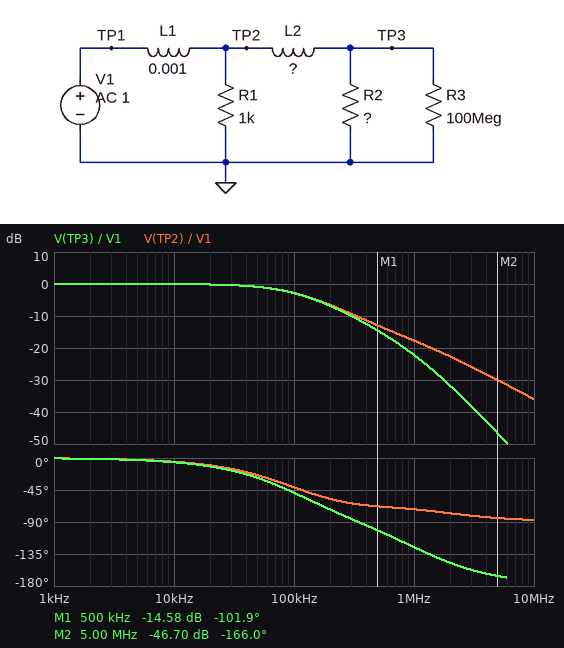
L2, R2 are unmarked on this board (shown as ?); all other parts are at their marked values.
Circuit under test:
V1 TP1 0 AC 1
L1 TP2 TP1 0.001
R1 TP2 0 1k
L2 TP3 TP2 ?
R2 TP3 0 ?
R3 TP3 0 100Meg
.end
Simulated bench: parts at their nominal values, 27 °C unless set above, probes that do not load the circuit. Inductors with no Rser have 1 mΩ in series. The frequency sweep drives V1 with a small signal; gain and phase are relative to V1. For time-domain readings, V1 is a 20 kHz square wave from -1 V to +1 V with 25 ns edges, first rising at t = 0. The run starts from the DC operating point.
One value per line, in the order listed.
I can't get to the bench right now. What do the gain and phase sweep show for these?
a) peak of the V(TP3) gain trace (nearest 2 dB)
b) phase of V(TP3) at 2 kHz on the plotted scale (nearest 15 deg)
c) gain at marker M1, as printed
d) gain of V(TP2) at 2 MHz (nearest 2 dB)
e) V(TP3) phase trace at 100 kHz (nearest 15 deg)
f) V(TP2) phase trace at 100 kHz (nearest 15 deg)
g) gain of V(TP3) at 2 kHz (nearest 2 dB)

0 dB
0 deg
-14.58 dB
-22 dB
-45 deg
-45 deg
0 dB
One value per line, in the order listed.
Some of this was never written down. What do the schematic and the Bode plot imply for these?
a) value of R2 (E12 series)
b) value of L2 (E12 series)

2.2 kΩ
470 µH
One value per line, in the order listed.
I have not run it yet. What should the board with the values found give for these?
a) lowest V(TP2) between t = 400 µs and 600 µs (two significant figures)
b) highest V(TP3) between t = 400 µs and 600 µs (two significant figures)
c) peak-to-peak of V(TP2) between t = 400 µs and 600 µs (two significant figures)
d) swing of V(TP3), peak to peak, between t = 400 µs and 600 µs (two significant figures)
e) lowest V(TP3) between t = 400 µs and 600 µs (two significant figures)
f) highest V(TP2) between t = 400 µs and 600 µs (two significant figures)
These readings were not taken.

-1.0 V
1.0 V
2.0 V
2.0 V
-1.0 V
1.0 V
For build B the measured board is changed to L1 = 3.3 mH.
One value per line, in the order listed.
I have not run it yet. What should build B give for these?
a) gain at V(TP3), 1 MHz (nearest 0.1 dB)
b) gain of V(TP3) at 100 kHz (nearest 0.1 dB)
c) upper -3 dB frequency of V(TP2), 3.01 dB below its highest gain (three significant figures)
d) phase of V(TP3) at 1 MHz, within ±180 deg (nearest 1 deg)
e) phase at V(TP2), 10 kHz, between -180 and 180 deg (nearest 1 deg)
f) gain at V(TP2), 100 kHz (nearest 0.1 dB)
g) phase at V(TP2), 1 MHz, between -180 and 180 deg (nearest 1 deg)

-32.3 dB
-10.2 dB
32.7 kHz
-130 deg
-17 deg
-10.1 dB
-77 deg
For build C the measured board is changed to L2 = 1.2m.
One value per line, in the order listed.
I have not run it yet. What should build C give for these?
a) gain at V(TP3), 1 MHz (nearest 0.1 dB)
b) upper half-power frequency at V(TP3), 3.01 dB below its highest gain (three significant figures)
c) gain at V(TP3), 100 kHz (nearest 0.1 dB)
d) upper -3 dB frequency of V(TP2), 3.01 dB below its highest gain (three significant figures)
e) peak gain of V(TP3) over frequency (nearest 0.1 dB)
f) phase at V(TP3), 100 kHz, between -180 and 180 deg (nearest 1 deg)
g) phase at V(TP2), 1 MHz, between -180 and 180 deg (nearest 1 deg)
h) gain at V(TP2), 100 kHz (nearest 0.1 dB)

-27.6 dB
91.8 kHz
-3.4 dB
102 kHz
0 dB
-58 deg
-75 deg
-2.9 dB
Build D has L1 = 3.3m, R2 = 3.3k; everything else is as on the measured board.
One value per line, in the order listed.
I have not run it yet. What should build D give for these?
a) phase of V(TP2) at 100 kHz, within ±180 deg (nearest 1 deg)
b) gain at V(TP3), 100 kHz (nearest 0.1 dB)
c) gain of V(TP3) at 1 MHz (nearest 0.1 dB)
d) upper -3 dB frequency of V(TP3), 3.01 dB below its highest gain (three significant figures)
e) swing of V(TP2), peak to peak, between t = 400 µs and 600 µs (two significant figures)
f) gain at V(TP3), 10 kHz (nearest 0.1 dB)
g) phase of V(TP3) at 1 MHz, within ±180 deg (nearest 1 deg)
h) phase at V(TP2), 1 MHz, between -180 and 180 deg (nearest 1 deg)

-69 deg
-9.3 dB
-30.4 dB
36.7 kHz
2.0 V
-0.3 dB
-122 deg
-80 deg
